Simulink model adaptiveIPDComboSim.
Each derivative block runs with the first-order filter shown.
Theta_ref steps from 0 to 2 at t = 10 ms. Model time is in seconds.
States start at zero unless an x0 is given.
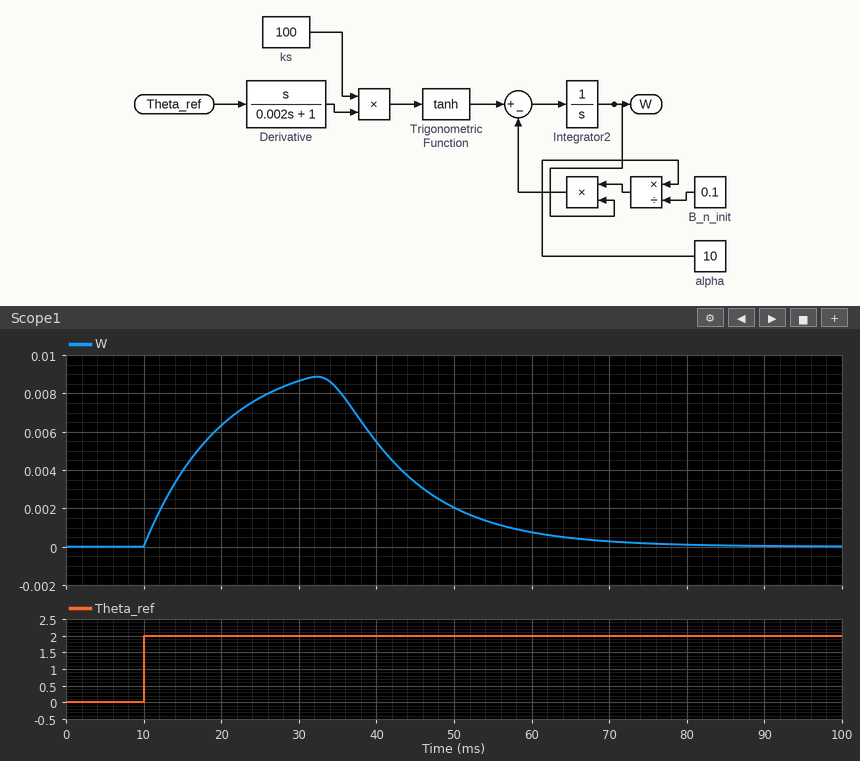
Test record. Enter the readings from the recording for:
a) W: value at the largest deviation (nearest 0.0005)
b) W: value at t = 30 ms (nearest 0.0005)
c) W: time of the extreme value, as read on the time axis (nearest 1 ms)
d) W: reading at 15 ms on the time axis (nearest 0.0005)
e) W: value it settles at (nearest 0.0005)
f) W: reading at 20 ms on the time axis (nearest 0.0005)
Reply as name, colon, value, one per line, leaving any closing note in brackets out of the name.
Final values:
W: value at the largest deviation: 0.0090
W: value at t = 30 ms: 0.0085
W: time of the extreme value, as read on the time axis: 32 ms
W: reading at 15 ms on the time axis: 0.0040
W: value it settles at: 0.0000
W: reading at 20 ms on the time axis: 0.0065
